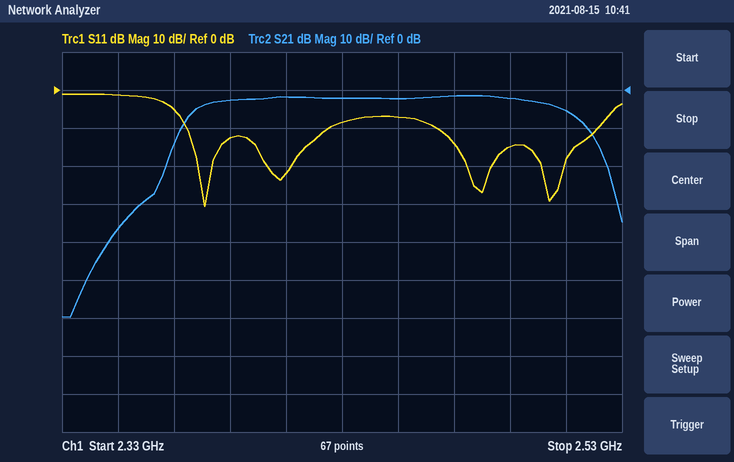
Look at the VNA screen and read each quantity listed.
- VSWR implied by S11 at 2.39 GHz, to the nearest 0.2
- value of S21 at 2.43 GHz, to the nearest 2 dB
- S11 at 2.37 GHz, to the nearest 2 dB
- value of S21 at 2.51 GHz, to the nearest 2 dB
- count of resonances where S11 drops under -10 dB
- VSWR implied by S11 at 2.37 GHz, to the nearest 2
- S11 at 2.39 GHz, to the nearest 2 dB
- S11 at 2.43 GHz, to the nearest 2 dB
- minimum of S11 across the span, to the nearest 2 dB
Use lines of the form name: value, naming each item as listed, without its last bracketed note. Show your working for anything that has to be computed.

VSWR implied by S11 at 2.39 GHz, to the nearest 0.2: |Γ| = 10^(-12/20) = 0.2512; VSWR = (1 + 0.2512)/(1 − 0.2512) ≈ 1.67, so 1.6 to the nearest 0.2
value of S21 at 2.43 GHz, to the nearest 2 dB: -2 dB
S11 at 2.37 GHz, to the nearest 2 dB: -6 dB
value of S21 at 2.51 GHz, to the nearest 2 dB: -6 dB
count of resonances where S11 drops under -10 dB: 4
VSWR implied by S11 at 2.37 GHz, to the nearest 2: |Γ| = 10^(-6/20) = 0.5012; VSWR = (1 + 0.5012)/(1 − 0.5012) ≈ 3.01, so 4 to the nearest 2
S11 at 2.39 GHz, to the nearest 2 dB: -12 dB
S11 at 2.43 GHz, to the nearest 2 dB: -8 dB
minimum of S11 across the span, to the nearest 2 dB: -30 dB
